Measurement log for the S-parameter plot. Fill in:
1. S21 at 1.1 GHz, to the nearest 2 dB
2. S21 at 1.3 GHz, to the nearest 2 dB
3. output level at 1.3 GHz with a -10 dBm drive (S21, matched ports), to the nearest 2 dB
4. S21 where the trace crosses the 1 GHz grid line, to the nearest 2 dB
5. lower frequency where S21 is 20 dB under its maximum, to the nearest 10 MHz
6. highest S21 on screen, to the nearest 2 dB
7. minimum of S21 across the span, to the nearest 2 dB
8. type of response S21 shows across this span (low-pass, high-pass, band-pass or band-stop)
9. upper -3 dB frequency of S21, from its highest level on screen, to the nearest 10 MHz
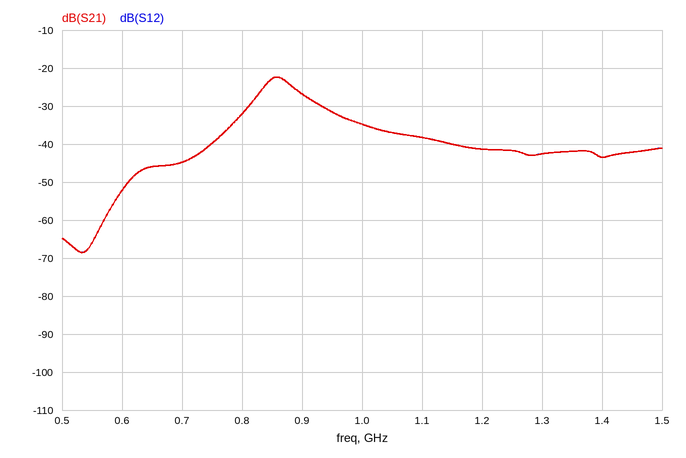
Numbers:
-38 dB
-42 dB
-52 dBm
-34 dB
730 MHz
-22 dB
-68 dB
band-pass
890 MHz
